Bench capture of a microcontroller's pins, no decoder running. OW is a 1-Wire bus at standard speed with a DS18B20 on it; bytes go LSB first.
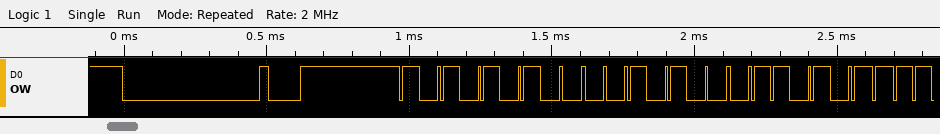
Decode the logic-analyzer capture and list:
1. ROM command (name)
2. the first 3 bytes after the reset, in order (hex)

Match ROM
55 28 D6
